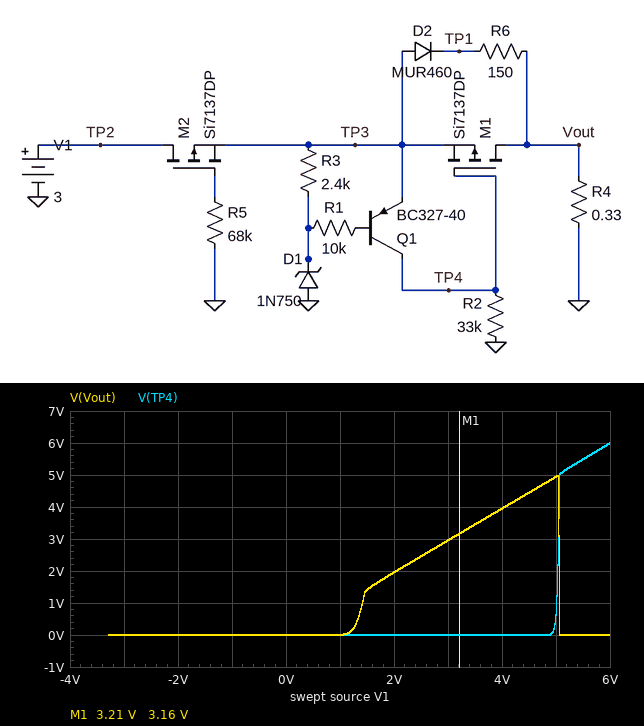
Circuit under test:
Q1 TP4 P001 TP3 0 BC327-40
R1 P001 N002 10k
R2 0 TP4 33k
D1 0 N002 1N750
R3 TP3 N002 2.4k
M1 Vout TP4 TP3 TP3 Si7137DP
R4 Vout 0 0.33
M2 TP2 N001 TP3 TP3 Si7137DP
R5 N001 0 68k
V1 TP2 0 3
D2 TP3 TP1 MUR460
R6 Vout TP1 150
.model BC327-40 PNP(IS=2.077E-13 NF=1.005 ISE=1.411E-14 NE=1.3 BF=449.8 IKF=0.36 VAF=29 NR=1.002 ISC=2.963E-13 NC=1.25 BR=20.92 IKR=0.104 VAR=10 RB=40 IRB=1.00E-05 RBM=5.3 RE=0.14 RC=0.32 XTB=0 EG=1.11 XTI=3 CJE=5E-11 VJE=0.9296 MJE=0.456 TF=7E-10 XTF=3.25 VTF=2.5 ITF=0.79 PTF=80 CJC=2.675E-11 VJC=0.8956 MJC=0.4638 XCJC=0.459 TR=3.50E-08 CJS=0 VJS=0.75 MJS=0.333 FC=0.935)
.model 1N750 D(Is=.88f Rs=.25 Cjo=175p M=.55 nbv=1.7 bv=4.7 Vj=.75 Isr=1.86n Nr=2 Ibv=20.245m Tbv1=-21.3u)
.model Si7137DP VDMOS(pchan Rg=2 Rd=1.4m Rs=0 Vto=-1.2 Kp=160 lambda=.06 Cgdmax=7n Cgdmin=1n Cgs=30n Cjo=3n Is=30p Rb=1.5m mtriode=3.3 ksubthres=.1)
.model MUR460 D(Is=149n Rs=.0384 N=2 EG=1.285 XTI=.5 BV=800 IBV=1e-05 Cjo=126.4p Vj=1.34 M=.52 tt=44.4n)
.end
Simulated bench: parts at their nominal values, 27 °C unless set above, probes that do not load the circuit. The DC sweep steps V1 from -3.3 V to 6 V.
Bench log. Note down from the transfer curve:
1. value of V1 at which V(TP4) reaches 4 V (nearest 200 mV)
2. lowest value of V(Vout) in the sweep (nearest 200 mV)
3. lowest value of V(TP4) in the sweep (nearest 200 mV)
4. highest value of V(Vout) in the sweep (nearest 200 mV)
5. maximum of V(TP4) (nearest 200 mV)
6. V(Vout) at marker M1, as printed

5.0 V
0 V
0 V
5.0 V
6.0 V
3.16 V
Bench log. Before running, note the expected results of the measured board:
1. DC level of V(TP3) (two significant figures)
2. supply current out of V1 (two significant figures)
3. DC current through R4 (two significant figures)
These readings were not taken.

3.0 V
9.0 A
9.0 A
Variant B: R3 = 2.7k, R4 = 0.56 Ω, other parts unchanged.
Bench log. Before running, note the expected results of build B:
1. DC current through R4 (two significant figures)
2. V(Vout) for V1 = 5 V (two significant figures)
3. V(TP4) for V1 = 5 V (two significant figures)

5.3 A
5.0 V
1.1 V
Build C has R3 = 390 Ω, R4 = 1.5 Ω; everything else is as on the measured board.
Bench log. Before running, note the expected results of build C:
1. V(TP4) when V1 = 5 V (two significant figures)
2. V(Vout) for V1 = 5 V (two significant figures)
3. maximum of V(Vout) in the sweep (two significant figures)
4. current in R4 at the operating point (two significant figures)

86 mV
5.0 V
5.1 V
2.0 A
